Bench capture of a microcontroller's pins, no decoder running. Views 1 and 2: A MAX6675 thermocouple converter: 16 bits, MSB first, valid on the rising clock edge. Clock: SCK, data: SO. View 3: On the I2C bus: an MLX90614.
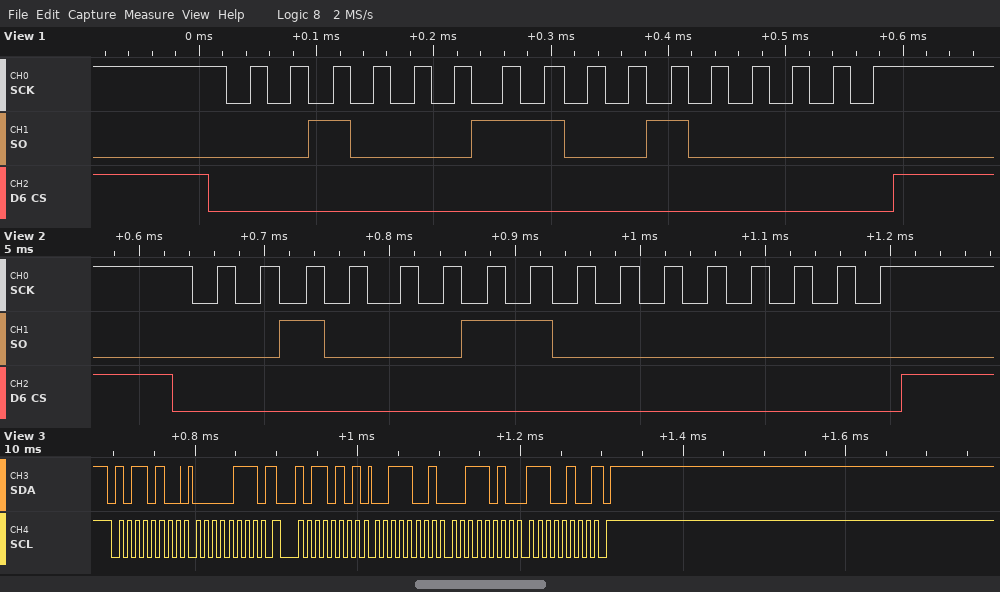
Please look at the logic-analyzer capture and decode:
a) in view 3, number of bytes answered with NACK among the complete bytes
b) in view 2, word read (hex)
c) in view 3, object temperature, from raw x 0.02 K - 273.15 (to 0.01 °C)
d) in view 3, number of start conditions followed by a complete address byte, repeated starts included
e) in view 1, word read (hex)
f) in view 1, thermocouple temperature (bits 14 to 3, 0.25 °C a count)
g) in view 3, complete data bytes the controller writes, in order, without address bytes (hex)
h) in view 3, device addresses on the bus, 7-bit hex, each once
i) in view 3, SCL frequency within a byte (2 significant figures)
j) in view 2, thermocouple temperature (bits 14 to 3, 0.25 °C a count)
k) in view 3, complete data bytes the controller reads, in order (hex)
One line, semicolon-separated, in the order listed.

1; 0x2300; 24.95 °C; 2; 0x2320; 281.00 °C; 07; 0x5A; 100 kHz; 280.00 °C; 39 3A E4
